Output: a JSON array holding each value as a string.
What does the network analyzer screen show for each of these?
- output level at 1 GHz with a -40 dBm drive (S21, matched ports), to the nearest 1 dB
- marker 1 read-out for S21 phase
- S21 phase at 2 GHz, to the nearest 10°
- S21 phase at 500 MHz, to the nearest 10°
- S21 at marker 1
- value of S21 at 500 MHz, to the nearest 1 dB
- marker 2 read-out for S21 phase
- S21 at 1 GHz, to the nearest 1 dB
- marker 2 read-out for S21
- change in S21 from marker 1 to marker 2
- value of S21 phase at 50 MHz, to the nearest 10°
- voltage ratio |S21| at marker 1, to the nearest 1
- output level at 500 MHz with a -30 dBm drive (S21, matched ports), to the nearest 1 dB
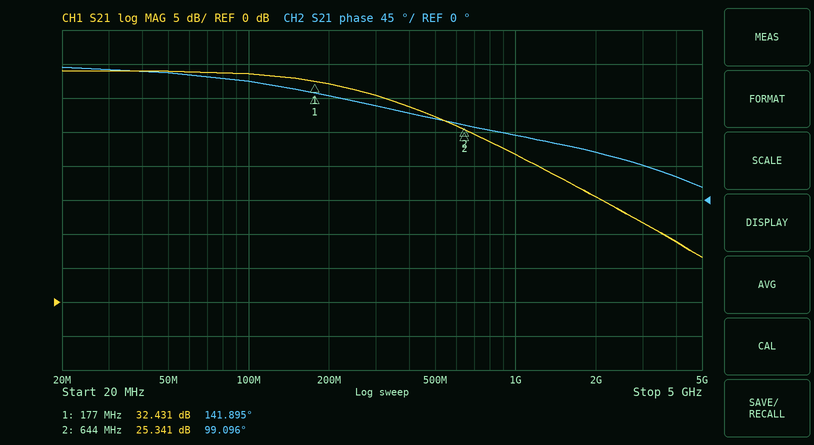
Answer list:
["-18 dBm", "141.895°", "60°", "110°", "32.431 dB", "27 dB", "99.096°", "22 dB", "25.341 dB", "-7.090 dB", "170°", "42", "-3 dBm"]
